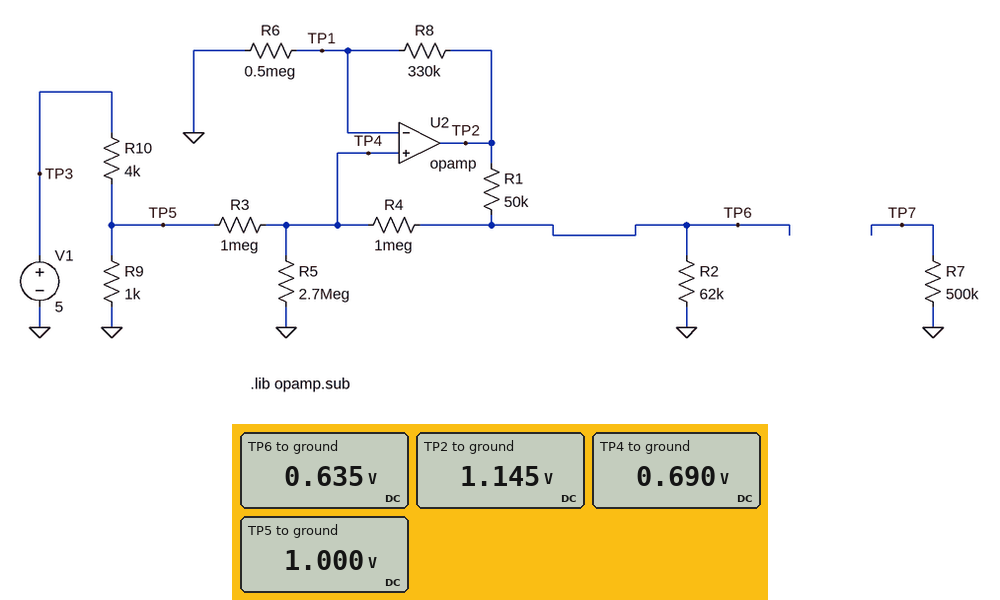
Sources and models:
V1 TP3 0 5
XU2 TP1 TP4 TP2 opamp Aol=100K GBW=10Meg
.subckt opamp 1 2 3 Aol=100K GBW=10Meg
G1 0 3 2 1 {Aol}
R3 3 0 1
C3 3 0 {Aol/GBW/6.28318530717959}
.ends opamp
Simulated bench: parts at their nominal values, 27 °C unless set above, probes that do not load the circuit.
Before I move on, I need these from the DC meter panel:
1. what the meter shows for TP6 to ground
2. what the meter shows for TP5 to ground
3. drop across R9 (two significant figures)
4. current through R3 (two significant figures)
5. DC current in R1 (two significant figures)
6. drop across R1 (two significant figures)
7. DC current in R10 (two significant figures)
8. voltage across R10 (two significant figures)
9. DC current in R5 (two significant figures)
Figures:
0.635 V
1.000 V
1.0 V
310 nA
10 µA
510 mV
1.0 mA
4.0 V
260 nA
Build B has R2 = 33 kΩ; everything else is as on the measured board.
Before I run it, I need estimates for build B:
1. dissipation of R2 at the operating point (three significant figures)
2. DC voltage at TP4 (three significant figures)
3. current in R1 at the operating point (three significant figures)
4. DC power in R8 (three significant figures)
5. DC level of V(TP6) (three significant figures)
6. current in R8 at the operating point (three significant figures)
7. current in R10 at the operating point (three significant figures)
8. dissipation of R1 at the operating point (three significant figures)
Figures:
4.64 µW
587 mV
11.7 µA
454 nW
391 mV
1.17 µA
1.00 mA
6.79 µW
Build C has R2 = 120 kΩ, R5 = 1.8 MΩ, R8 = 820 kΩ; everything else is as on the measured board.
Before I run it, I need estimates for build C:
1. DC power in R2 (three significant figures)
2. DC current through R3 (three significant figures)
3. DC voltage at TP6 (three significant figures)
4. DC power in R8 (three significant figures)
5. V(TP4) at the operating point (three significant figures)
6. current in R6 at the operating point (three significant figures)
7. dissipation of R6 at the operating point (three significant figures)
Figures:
53.9 µW
386 nA
2.54 V
6.30 µW
1.39 V
2.77 µA
3.84 µW
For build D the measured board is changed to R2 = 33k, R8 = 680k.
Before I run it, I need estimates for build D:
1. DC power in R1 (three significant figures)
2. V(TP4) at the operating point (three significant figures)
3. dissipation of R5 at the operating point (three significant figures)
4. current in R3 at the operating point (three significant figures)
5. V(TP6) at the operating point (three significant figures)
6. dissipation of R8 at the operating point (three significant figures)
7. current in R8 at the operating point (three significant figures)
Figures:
19.7 µW
699 mV
181 nW
301 nA
656 mV
1.33 µW
1.40 µA
